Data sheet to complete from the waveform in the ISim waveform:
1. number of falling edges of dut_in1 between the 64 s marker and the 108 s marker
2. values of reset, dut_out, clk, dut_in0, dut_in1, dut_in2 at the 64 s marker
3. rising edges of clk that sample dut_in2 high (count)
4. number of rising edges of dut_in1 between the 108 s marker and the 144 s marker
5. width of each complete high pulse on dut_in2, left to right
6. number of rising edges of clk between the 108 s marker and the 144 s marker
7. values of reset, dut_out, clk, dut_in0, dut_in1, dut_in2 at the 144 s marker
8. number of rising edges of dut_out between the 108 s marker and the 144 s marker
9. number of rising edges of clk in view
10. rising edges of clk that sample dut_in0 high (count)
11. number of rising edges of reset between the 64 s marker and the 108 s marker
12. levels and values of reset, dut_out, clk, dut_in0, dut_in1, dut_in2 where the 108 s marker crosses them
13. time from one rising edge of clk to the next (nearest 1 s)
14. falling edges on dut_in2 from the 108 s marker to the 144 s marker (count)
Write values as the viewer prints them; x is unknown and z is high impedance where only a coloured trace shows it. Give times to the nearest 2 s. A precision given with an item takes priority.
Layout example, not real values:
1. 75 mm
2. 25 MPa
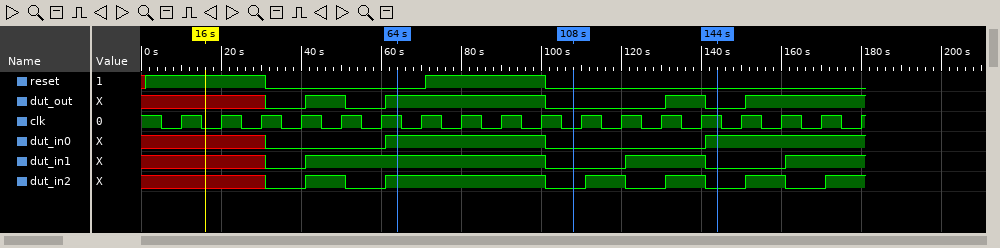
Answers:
1. 1
2. reset=0, dut_out=1, clk=1, dut_in0=1, dut_in1=1, dut_in2=1
3. 9
4. 1
5. 10 s, 40 s, 10 s, 10 s, 10 s
6. 4
7. reset=0, dut_out=0, clk=1, dut_in0=1, dut_in1=0, dut_in2=0
8. 1
9. 18
10. 8
11. 1
12. reset=0, dut_out=0, clk=0, dut_in0=0, dut_in1=0, dut_in2=0
13. 10 s
14. 2
